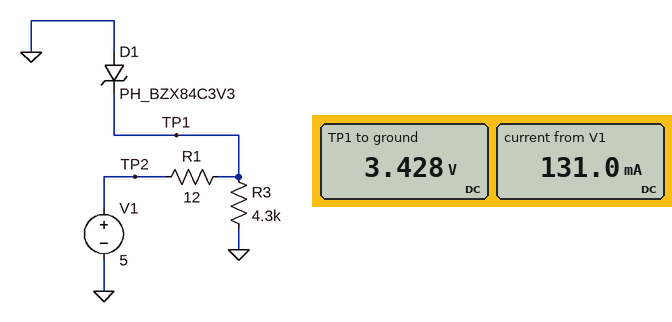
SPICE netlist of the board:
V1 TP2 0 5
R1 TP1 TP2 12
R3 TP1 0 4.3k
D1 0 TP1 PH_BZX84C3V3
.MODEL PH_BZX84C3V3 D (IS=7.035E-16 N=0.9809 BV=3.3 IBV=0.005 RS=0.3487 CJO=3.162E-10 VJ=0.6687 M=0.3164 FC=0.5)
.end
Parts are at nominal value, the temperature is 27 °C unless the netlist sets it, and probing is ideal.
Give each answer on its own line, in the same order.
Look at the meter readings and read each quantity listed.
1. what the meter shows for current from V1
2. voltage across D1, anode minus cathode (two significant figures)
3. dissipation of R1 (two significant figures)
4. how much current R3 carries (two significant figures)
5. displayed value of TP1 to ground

131.0 mA
-3.4 V
210 mW
800 µA
3.428 V
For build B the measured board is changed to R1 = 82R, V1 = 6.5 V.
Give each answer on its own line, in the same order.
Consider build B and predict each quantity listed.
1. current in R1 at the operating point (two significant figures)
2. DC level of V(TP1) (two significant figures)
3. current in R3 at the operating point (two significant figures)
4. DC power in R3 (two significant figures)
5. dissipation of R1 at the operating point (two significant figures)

38 mA
3.4 V
780 µA
2.6 mW
120 mW
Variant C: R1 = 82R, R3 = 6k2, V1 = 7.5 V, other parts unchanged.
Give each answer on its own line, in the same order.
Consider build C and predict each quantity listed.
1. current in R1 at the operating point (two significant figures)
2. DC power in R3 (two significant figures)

50 mA
1.8 mW
